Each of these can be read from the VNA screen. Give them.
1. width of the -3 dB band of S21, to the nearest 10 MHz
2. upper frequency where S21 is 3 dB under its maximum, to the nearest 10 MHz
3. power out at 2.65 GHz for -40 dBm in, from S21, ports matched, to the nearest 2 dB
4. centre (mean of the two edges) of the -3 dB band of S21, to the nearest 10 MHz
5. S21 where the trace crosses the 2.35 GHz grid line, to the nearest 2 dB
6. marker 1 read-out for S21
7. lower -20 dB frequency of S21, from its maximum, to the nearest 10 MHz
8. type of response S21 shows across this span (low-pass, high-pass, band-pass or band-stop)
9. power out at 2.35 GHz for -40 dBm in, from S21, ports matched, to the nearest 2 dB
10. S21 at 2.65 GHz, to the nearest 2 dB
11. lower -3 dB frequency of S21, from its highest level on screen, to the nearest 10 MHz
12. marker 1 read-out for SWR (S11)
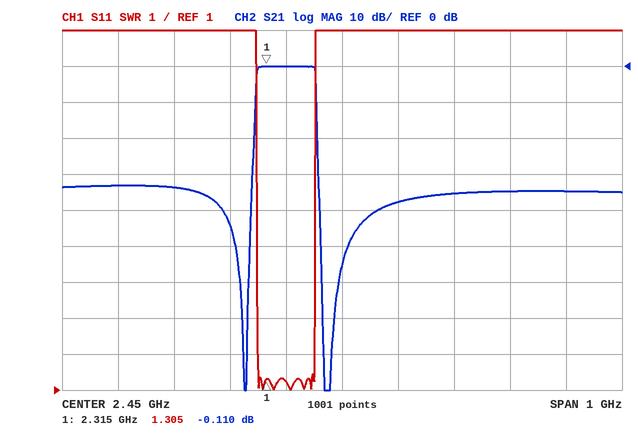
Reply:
100 MHz
2.40 GHz
-76 dBm
2.35 GHz
0 dB
-0.110 dB
2.29 GHz
band-pass
-40 dBm
-36 dB
2.30 GHz
1.305
